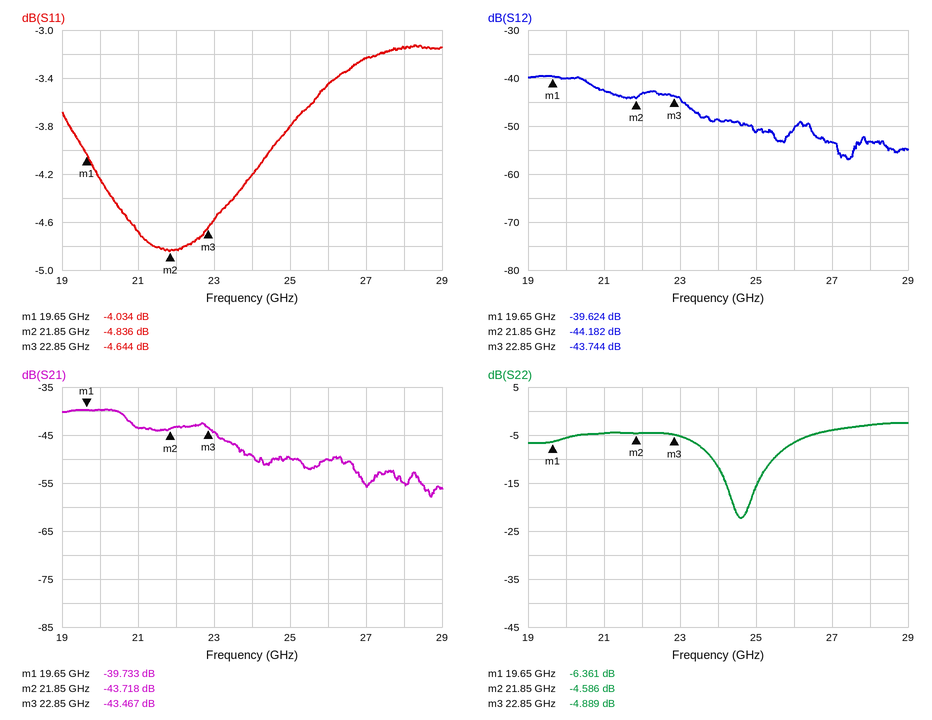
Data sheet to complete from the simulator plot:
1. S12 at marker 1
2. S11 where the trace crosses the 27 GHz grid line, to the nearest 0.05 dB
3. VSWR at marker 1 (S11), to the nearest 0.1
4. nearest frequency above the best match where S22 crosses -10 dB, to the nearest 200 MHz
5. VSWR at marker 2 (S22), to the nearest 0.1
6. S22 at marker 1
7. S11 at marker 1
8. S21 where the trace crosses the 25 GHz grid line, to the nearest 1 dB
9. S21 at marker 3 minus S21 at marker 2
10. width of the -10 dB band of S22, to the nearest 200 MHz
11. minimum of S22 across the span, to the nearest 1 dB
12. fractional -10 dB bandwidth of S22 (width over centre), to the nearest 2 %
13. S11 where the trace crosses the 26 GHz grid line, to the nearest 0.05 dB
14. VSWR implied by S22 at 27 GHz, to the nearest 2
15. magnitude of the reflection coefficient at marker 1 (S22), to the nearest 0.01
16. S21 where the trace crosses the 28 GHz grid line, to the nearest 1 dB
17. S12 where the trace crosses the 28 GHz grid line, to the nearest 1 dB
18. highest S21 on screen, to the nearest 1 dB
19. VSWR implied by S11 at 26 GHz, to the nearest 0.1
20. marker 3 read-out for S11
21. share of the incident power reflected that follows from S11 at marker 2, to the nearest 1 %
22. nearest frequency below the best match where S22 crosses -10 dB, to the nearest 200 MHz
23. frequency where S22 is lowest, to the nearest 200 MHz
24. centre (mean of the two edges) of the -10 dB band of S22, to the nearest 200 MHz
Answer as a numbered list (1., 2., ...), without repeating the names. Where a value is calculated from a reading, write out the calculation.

1. -39.624 dB
2. -3.25 dB
3. (1 + 0.6285)/(1 − 0.6285) ≈ 4.4
4. 25.4 GHz
5. (1 + 0.5898)/(1 − 0.5898) ≈ 3.9
6. -6.361 dB
7. -4.034 dB
8. -50 dB
9. -43.467 − (-43.718) = 0.251 dB
10. 25.4 GHz − 23.8 GHz = 1.6 GHz
11. -22 dB
12. 1.6 GHz / 24.6 GHz ≈ 6 %
13. -3.45 dB
14. |Γ| = 10^(-4/20) = 0.6310; VSWR = (1 + 0.6310)/(1 − 0.6310) ≈ 4
15. 10^(-6.361/20) ≈ 0.48
16. -55 dB
17. -53 dB
18. -40 dB
19. |Γ| = 10^(-3.45/20) = 0.6722; VSWR = (1 + 0.6722)/(1 − 0.6722) ≈ 5.1
20. -4.644 dB
21. 10^(-4.836/10) ≈ 33 %
22. 23.8 GHz
23. 24.6 GHz
24. 24.6 GHz
